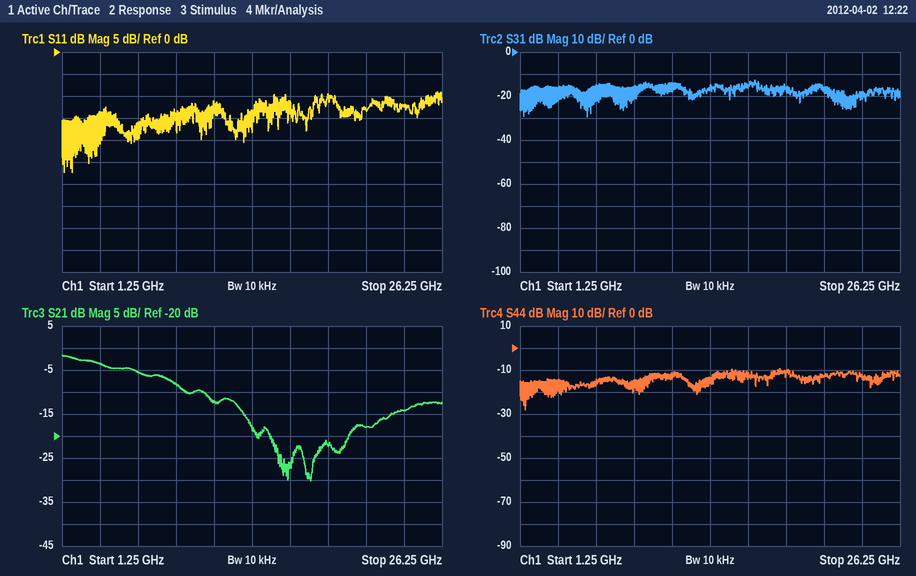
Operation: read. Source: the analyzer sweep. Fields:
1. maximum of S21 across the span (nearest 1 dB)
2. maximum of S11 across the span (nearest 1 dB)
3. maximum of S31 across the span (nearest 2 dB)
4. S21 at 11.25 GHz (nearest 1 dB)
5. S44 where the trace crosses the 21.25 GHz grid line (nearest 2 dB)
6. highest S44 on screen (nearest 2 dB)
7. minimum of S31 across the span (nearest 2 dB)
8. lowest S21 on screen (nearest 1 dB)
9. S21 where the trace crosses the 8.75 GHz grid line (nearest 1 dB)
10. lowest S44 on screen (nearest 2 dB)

-2 dB
-9 dB
-12 dB
-12 dB
-12 dB
-10 dB
-30 dB
-30 dB
-8 dB
-28 dB
